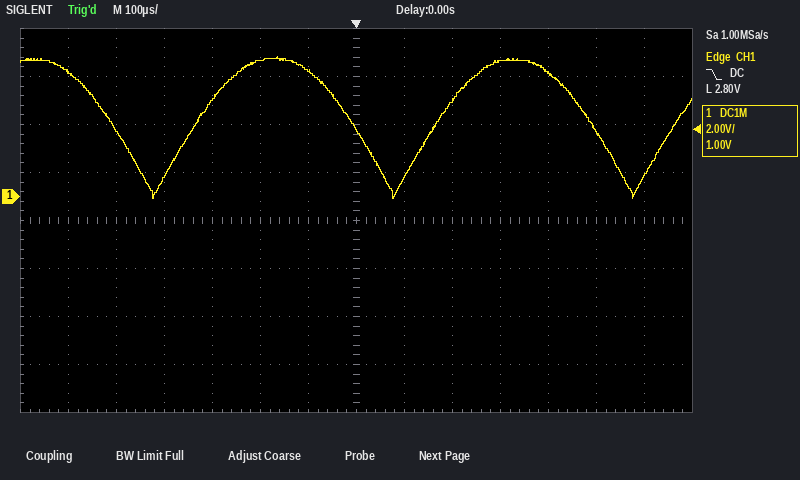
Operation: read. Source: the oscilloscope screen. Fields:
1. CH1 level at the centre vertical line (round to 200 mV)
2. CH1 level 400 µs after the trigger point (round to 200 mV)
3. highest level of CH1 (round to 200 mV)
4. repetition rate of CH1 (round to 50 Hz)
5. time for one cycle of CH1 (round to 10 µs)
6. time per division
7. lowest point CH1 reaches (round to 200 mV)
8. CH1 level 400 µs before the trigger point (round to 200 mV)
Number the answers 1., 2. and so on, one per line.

1. 2.8 V
2. 5.2 V
3. 5.8 V
4. 2.00 kHz
5. 500 µs
6. 100 µs
7. 0.0 V
8. 800 mV
